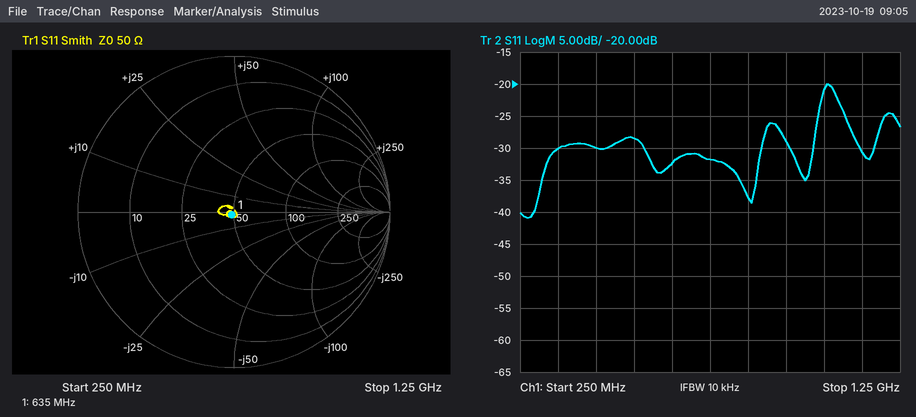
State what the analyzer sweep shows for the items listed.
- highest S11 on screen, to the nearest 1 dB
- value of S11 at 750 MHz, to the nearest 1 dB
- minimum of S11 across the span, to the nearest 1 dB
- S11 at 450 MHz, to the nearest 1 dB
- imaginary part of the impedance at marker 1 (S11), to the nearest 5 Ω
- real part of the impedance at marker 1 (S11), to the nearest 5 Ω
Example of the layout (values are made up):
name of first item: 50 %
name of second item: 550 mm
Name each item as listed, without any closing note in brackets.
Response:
highest S11 on screen, to the nearest 1 dB: -20 dB
value of S11 at 750 MHz, to the nearest 1 dB: -32 dB
minimum of S11 across the span, to the nearest 1 dB: -41 dB
S11 at 450 MHz, to the nearest 1 dB: -30 dB
imaginary part of the impedance at marker 1 (S11), to the nearest 5 Ω: 0 Ω
real part of the impedance at marker 1 (S11), to the nearest 5 Ω: 50 Ω
